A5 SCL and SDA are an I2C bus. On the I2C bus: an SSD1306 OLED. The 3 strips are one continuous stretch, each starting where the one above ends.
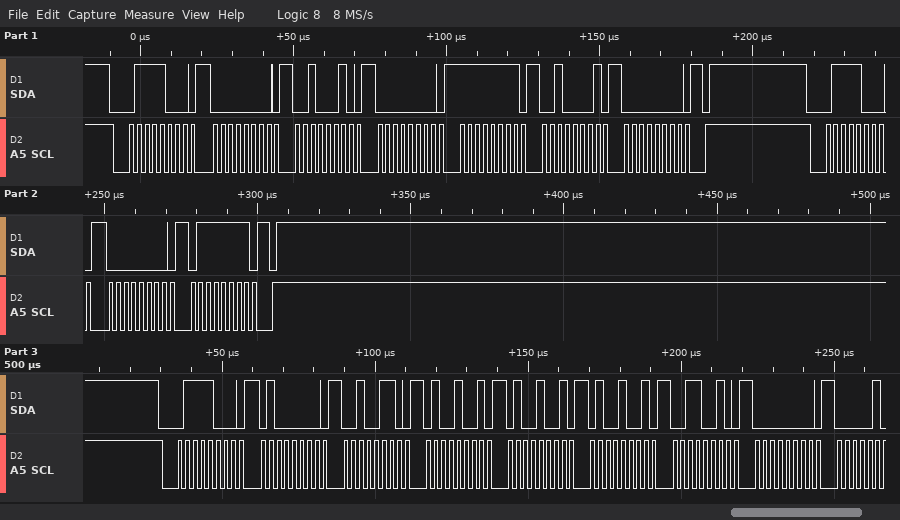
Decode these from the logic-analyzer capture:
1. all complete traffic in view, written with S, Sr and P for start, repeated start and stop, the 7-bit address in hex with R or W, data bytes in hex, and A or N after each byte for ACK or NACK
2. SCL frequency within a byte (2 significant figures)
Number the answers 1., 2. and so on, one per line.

1. S 3CW A 00 A 22 A 00 A FF A 21 A 00 A P S 3CW A 00 A 7F A P S 3CW A 40 A 26 A 49 A 49 A 49 A 32 A 00 A
2. 400 kHz
